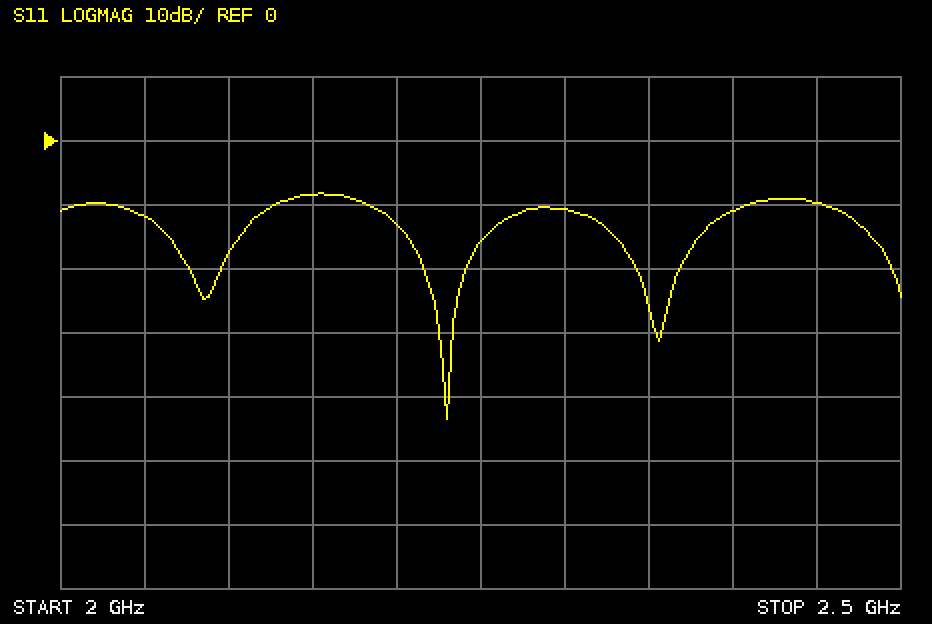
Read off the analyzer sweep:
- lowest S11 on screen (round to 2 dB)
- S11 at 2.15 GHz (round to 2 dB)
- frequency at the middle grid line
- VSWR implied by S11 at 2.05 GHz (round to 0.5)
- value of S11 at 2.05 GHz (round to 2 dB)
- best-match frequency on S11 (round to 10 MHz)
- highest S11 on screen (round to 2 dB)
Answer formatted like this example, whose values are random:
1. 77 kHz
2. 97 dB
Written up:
1. -44 dB
2. -8 dB
3. 2.25 GHz
4. 1.5
5. -12 dB
6. 2.23 GHz
7. -8 dB
